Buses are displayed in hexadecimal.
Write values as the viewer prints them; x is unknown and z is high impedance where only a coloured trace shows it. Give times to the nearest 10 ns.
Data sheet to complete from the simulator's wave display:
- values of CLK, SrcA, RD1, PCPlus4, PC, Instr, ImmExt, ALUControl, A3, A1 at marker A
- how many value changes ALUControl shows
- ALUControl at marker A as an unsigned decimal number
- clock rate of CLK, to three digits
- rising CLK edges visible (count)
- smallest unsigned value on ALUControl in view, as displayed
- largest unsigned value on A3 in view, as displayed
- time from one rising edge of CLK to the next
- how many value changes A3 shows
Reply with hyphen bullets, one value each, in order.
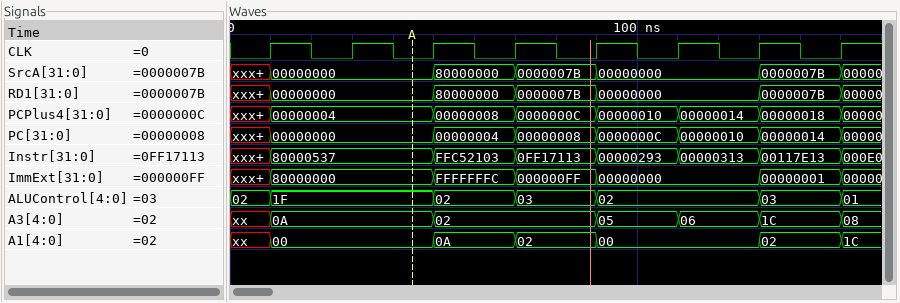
- CLK=0, SrcA=00000000, RD1=00000000, PCPlus4=00000004, PC=00000000, Instr=80000537, ImmExt=80000000, ALUControl=1F, A3=0A, A1=00
- 6
- 31
- 50.0 MHz
- 8
- 01
- 1C
- 20 ns
- 6
